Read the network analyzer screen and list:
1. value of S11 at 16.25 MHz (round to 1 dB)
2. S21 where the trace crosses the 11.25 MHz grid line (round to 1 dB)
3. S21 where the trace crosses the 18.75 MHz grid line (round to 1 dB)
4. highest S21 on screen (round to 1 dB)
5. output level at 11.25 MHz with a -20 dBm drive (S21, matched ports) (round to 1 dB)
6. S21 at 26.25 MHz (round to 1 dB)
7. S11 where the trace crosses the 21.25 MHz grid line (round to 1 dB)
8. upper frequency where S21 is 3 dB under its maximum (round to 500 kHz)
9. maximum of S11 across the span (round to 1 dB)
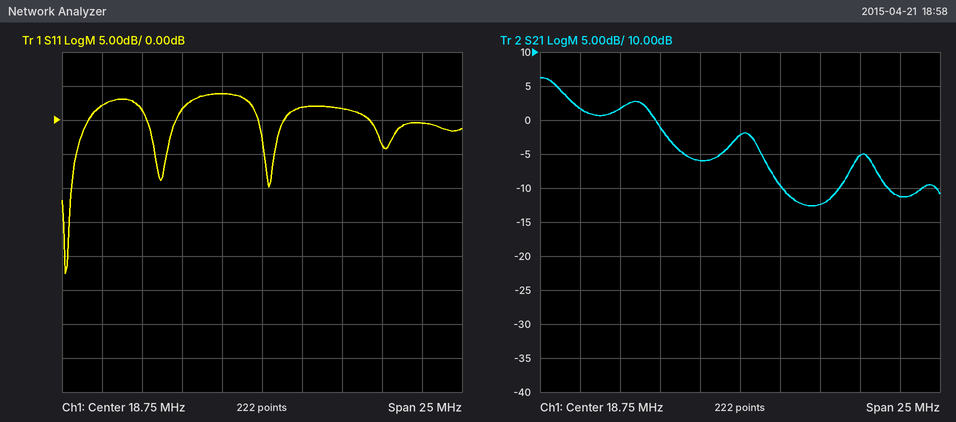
4 dB
2 dB
-2 dB
6 dB
-18 dBm
-5 dB
2 dB
8.0 MHz
4 dB
